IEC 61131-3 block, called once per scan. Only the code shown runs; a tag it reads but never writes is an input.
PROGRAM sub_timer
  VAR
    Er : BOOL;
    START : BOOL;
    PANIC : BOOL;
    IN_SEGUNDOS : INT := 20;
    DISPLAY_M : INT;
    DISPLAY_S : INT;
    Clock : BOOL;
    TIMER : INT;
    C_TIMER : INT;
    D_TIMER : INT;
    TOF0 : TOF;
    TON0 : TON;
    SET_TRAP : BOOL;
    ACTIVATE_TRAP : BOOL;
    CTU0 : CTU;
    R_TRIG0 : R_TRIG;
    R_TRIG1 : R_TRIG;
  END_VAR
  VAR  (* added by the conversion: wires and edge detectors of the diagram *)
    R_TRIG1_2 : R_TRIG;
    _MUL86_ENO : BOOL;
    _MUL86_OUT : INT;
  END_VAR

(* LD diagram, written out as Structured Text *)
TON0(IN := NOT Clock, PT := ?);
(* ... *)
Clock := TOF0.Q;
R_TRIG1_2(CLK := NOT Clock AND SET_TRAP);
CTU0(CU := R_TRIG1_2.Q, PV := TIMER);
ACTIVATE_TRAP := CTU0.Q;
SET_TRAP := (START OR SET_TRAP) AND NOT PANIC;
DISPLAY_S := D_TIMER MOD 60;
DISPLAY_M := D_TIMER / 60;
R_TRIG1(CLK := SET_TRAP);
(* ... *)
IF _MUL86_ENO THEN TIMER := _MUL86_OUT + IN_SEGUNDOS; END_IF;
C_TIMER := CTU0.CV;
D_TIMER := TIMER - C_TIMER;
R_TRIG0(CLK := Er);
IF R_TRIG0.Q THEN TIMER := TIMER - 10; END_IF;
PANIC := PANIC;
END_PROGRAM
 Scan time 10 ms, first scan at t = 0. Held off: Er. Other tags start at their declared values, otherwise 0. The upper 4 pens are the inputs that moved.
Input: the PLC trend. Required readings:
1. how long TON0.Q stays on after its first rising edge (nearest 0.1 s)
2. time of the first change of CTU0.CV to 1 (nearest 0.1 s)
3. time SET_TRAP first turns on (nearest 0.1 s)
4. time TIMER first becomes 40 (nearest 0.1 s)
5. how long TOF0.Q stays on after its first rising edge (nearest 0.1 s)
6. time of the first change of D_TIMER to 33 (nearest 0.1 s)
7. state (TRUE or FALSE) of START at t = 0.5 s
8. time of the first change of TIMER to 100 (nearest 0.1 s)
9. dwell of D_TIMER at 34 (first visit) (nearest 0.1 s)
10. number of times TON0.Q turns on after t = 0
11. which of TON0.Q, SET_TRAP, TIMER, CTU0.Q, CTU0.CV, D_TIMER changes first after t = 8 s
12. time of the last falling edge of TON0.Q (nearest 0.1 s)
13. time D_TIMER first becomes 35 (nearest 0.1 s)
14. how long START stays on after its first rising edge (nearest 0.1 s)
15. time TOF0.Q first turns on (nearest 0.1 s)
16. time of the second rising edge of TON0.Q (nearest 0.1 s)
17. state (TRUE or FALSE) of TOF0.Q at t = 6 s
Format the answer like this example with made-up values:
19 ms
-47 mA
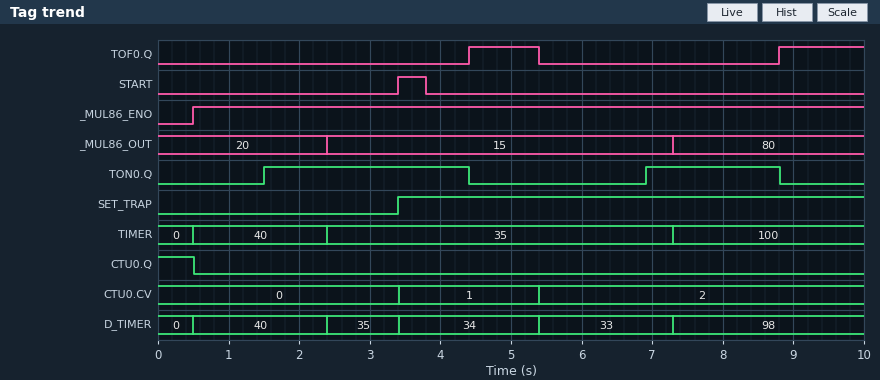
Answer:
2.9 s
3.4 s
3.4 s
0.5 s
1.0 s
5.4 s
FALSE
7.3 s
2.0 s
2
TON0.Q
8.8 s
2.4 s
0.4 s
4.4 s
6.9 s
FALSE
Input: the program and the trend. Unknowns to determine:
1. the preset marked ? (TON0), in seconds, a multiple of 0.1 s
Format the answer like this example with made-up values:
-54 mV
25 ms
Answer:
1.5 s
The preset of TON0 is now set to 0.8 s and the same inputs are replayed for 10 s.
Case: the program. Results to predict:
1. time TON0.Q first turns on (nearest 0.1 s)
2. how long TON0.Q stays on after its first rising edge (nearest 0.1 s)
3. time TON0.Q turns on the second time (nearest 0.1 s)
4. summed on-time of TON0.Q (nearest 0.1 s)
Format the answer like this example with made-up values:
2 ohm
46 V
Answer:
0.8 s
3.6 s
6.2 s
6.2 s
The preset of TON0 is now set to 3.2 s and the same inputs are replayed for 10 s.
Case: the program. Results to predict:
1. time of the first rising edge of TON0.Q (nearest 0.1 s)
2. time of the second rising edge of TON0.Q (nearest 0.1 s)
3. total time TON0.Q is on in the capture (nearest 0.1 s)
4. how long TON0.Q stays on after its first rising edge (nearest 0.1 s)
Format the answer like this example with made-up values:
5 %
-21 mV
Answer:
3.2 s
8.6 s
1.4 s
1.2 s
